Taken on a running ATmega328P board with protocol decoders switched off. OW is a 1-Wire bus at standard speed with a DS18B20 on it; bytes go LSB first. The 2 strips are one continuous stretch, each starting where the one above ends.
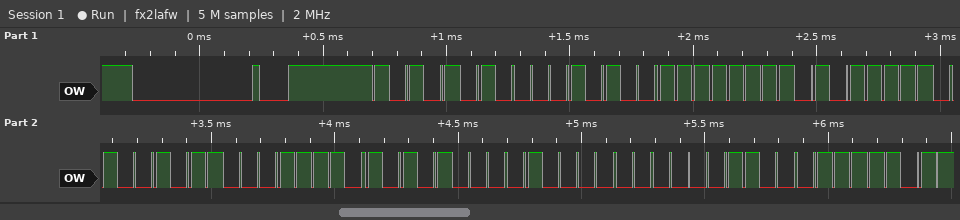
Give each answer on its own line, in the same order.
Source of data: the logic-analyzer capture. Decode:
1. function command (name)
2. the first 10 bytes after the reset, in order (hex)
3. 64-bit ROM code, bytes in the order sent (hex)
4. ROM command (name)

Read Scratchpad
55 28 FF FA D2 78 15 02 30 BE
28 FF FA D2 78 15 02 30
Match ROM
